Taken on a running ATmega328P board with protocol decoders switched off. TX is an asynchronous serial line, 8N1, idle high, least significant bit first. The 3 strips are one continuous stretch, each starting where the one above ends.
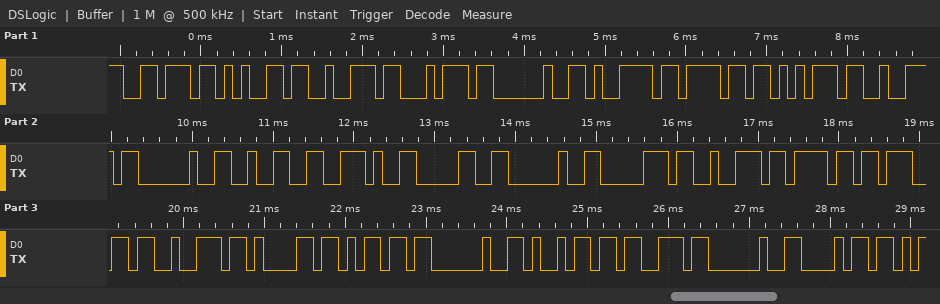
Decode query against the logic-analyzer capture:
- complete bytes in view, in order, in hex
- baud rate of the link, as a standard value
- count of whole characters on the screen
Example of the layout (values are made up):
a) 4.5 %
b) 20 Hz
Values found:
a) 76 65 72 74 20 79 6F 75 72 20 32 2E 30 20 70 72 6F 67 72 61 6D 20 69 73 20 68
b) 9600 baud
c) 26
